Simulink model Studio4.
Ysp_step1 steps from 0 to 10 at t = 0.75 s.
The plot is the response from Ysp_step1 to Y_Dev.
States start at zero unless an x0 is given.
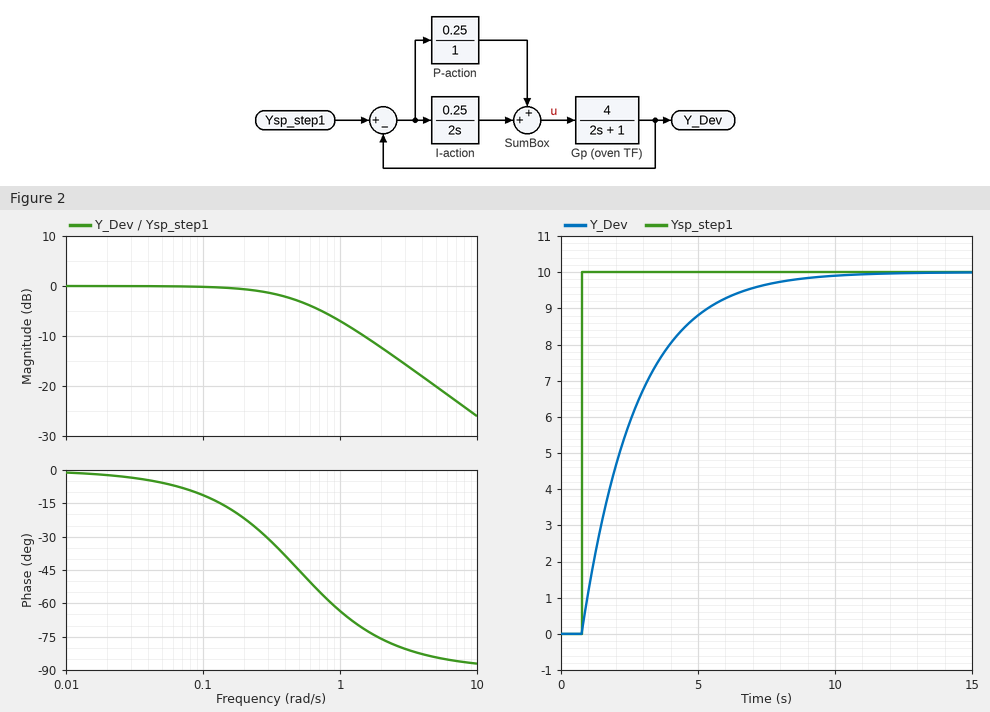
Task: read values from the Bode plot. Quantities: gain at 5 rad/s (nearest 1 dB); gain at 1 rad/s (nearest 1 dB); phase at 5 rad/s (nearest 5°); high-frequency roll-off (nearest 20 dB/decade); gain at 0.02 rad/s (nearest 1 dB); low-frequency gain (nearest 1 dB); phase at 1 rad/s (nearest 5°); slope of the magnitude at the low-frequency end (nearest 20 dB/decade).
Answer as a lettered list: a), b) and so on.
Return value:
a) -20 dB
b) -7 dB
c) -85°
d) -20 dB/decade
e) 0 dB
f) 0 dB
g) -65°
h) 0 dB/decade
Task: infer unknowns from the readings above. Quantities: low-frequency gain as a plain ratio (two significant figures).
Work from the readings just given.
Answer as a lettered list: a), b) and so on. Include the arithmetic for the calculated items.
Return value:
a) 10^(0 / 20) = 1.0
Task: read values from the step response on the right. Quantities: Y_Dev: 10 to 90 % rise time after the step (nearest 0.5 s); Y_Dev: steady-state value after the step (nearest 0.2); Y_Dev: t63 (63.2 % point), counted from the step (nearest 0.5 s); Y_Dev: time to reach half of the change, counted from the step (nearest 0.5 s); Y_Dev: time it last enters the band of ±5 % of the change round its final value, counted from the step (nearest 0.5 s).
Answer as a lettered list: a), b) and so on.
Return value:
a) 4.5 s
b) 10.0
c) 2.0 s
d) 1.5 s
e) 6.0 s
